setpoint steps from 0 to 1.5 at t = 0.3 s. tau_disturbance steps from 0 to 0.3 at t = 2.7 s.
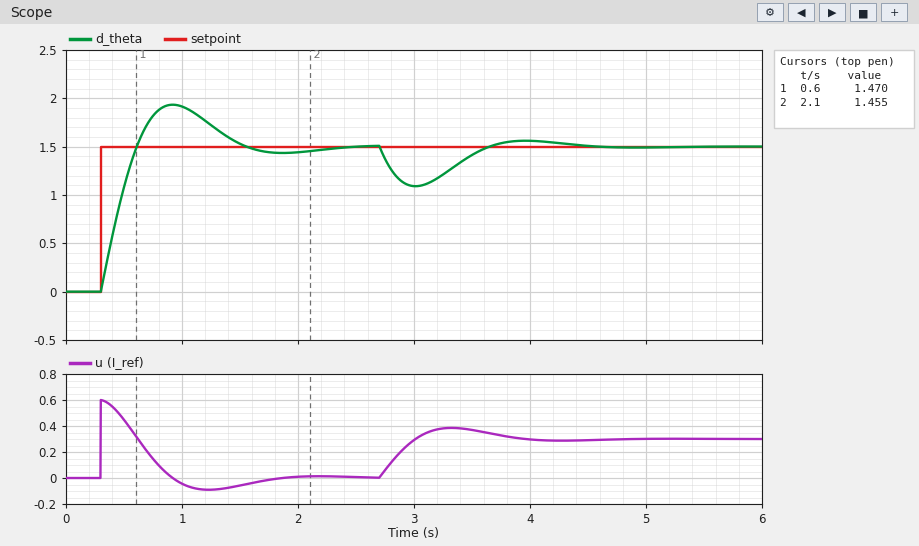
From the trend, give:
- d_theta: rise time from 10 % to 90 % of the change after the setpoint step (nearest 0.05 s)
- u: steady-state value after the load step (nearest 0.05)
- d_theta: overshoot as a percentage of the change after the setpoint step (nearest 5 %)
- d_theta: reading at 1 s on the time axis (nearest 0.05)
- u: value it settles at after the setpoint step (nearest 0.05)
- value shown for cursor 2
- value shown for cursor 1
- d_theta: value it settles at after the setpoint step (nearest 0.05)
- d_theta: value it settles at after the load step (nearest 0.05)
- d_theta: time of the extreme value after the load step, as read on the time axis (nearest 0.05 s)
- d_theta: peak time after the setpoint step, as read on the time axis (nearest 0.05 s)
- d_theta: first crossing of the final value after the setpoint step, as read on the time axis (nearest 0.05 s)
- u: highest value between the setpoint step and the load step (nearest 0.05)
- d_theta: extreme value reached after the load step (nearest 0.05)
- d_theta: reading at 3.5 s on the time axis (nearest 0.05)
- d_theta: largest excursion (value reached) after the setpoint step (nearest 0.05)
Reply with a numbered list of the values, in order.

1. 0.25 s
2. 0.30
3. 30 %
4. 1.90
5. 0.00
6. 1.455
7. 1.470
8. 1.50
9. 1.50
10. 3.00 s
11. 0.90 s
12. 0.60 s
13. 0.60
14. 1.10
15. 1.40
16. 1.95
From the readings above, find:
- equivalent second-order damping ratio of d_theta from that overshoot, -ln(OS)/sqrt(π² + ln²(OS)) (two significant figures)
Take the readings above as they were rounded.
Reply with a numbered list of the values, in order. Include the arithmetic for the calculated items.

1. ln(0.3) = -1.204; 1.204 / sqrt(9.870 + 1.450) = 0.36
